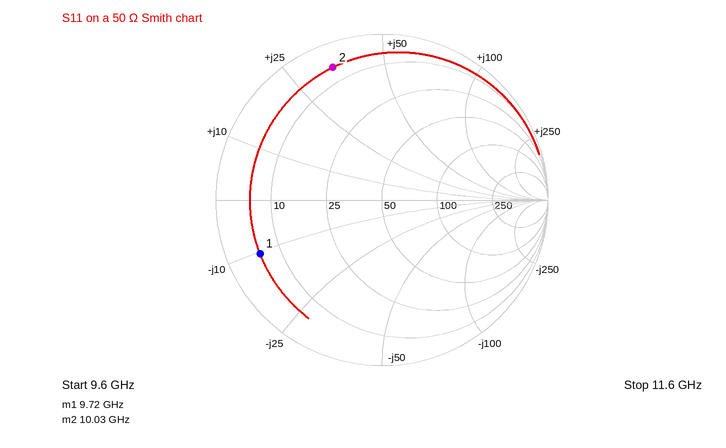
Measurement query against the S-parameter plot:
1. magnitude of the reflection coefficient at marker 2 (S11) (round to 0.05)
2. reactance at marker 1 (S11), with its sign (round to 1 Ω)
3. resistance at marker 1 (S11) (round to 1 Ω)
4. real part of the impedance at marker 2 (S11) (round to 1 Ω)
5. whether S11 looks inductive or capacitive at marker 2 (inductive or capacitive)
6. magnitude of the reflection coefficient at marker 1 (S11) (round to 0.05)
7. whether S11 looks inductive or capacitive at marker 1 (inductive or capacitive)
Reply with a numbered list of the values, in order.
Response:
1. 0.85
2. -10 Ω
3. 6 Ω
4. 6 Ω
5. inductive
6. 0.80
7. capacitive
